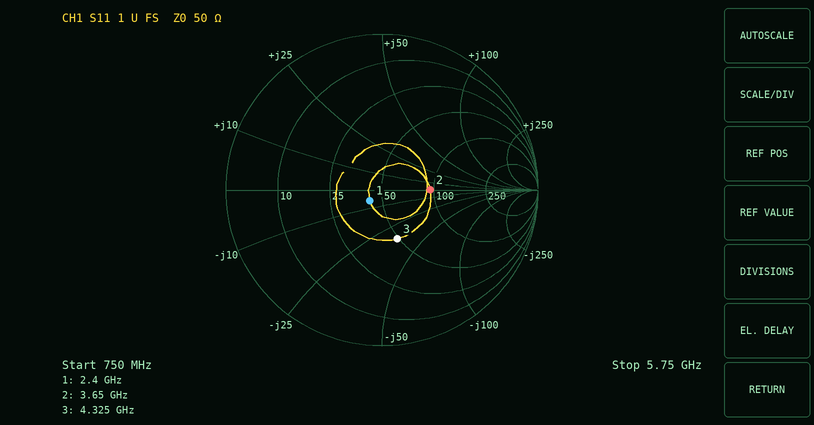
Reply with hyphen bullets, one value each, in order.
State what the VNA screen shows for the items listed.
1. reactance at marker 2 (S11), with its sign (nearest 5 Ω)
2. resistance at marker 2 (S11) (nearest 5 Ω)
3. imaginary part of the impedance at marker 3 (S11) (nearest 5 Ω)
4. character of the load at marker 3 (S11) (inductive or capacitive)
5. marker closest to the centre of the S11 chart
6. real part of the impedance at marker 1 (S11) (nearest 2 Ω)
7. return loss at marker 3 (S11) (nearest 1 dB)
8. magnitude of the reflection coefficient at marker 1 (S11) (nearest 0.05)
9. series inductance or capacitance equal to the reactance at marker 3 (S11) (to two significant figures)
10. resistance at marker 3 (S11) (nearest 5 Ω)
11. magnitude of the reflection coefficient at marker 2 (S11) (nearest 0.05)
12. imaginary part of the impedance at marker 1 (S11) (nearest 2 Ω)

- 0 Ω
- 95 Ω
- -35 Ω
- capacitive
- marker 1
- 42 Ω
- 10 dB
- 0.10
- 1.1 pF
- 50 Ω
- 0.30
- -6 Ω
